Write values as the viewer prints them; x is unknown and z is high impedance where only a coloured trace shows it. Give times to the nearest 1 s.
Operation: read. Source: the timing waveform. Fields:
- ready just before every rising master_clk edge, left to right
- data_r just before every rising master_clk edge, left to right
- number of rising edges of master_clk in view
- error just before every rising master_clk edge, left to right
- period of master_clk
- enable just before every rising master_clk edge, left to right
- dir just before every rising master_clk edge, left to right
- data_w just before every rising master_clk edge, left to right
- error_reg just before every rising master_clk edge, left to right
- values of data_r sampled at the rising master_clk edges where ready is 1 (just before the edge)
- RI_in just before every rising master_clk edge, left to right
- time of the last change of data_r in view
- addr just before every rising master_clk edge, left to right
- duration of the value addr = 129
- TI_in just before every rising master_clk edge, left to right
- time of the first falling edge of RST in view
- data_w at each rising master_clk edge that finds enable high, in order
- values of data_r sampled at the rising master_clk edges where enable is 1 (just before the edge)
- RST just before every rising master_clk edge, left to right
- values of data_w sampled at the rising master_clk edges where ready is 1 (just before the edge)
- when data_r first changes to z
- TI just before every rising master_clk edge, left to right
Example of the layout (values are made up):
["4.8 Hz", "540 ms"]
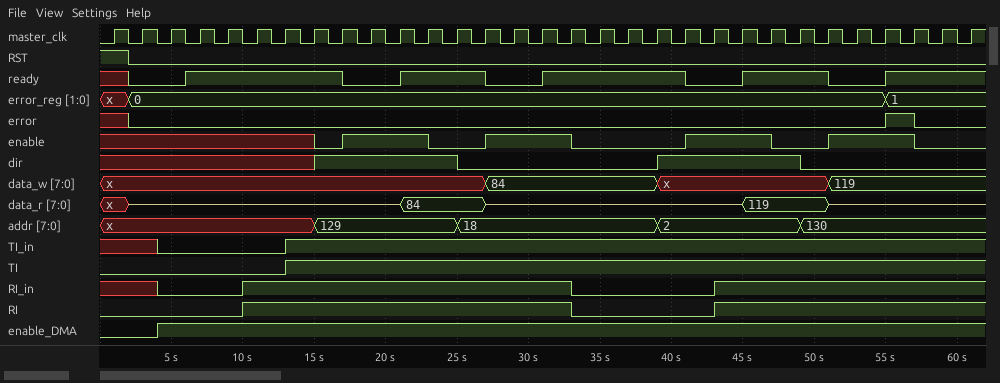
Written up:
["x 0 0 1 1 1 1 1 1 0 0 1 1 1 0 0 1 1 1 1 1 0 0 1 1 1 0 0 1 1 1", "x, z, z, z, z, z, z, z, z, z, z, 84, 84, 84, z, z, z, z, z, z, z, z, z, 119, 119, 119, z, z, z, z, z", "31", "x 0 0 0 0 0 0 0 0 0 0 0 0 0 0 0 0 0 0 0 0 0 0 0 0 0 0 0 1 0 0", "2 s", "x x x x x x x x 0 1 1 1 0 0 1 1 1 0 0 0 0 1 1 1 0 0 1 1 1 0 0", "x x x x x x x x 1 1 1 1 1 0 0 0 0 0 0 0 1 1 1 1 1 0 0 0 0 0 0", "x, x, x, x, x, x, x, x, x, x, x, x, x, x, 84, 84, 84, 84, 84, 84, x, x, x, x, x, x, 119, 119, 119, 119, 119", "x, 0, 0, 0, 0, 0, 0, 0, 0, 0, 0, 0, 0, 0, 0, 0, 0, 0, 0, 0, 0, 0, 0, 0, 0, 0, 0, 0, 1, 1, 1", "z, z, z, z, z, z, 84, 84, 84, z, z, z, z, z, 119, 119, 119, z, z, z", "x x 0 0 0 1 1 1 1 1 1 1 1 1 1 1 1 0 0 0 0 0 1 1 1 1 1 1 1 1 1", "51 s", "x, x, x, x, x, x, x, x, 129, 129, 129, 129, 129, 18, 18, 18, 18, 18, 18, 18, 2, 2, 2, 2, 2, 130, 130, 130, 130, 130, 130", "10 s", "x x 0 0 0 0 0 1 1 1 1 1 1 1 1 1 1 1 1 1 1 1 1 1 1 1 1 1 1 1 1", "2 s", "x, x, x, 84, 84, 84, x, x, x, 119, 119, 119", "z, z, 84, z, z, z, z, z, 119, z, z, z", "1 0 0 0 0 0 0 0 0 0 0 0 0 0 0 0 0 0 0 0 0 0 0 0 0 0 0 0 0 0 0", "x, x, x, x, x, x, x, x, x, 84, 84, 84, 84, x, x, x, x, 119, 119, 119", "2 s", "0 0 0 0 0 0 0 1 1 1 1 1 1 1 1 1 1 1 1 1 1 1 1 1 1 1 1 1 1 1 1"]
